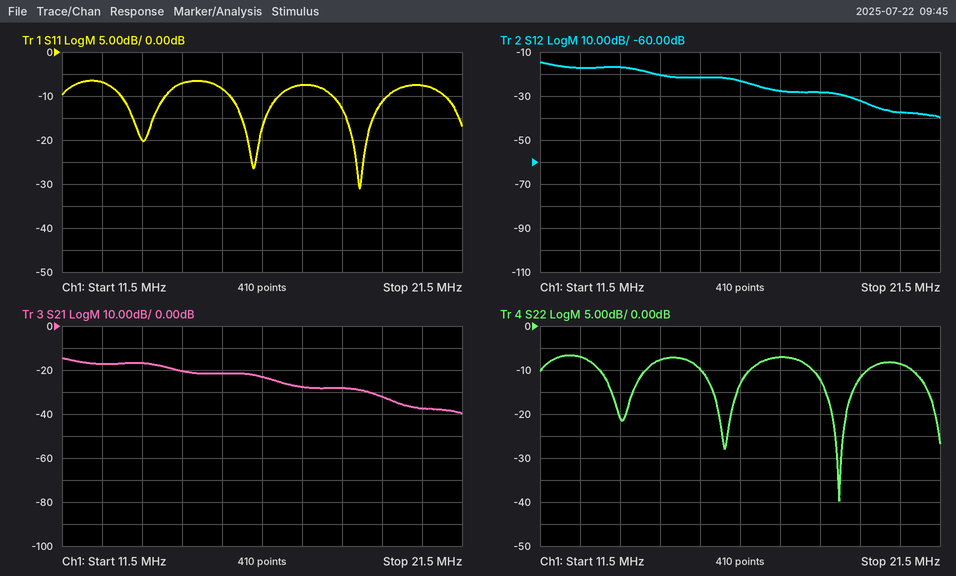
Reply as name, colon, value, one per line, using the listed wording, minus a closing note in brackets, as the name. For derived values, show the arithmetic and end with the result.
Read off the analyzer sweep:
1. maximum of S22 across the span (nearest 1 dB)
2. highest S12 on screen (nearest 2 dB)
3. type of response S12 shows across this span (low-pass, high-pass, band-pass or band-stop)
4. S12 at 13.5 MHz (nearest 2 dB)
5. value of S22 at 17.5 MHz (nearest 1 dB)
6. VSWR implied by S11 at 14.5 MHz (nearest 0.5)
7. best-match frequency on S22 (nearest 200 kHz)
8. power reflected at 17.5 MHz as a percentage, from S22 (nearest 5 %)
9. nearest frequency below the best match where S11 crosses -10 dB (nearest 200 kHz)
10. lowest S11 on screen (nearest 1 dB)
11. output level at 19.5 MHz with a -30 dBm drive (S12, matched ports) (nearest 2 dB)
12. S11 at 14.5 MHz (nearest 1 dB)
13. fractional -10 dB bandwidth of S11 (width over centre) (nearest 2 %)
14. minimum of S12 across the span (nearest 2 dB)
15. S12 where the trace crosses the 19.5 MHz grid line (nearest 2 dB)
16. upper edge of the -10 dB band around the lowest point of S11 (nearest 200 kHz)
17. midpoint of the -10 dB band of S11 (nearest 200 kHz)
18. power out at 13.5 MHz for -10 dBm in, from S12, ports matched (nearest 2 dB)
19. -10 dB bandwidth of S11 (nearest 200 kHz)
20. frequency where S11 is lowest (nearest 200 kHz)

maximum of S22 across the span: -7 dB
highest S12 on screen: -14 dB
type of response S12 shows across this span: low-pass
S12 at 13.5 MHz: -16 dB
value of S22 at 17.5 MHz: -7 dB
VSWR implied by S11 at 14.5 MHz: |Γ| = 10^(-7/20) = 0.4467; VSWR = (1 + 0.4467)/(1 − 0.4467) ≈ 2.61, so 2.5 to the nearest 0.5
best-match frequency on S22: 19.0 MHz
power reflected at 17.5 MHz as a percentage, from S22: 10^(-7/10) ≈ 20 %
nearest frequency below the best match where S11 crosses -10 dB: 18.2 MHz
lowest S11 on screen: -31 dB
output level at 19.5 MHz with a -30 dBm drive (S12, matched ports): -30 dBm + (-32 dB) = -62 dBm
S11 at 14.5 MHz: -7 dB
fractional -10 dB bandwidth of S11 (width over centre): 1.4 MHz / 18.9 MHz ≈ 7.41 %, so 8 % to the nearest 2 %
minimum of S12 across the span: -40 dB
S12 where the trace crosses the 19.5 MHz grid line: -32 dB
upper edge of the -10 dB band around the lowest point of S11: 19.6 MHz
midpoint of the -10 dB band of S11: 19.0 MHz
power out at 13.5 MHz for -10 dBm in, from S12, ports matched: -10 dBm + (-16 dB) = -26 dBm
-10 dB bandwidth of S11: 19.6 MHz − 18.2 MHz = 1.4 MHz
frequency where S11 is lowest: 19.0 MHz
